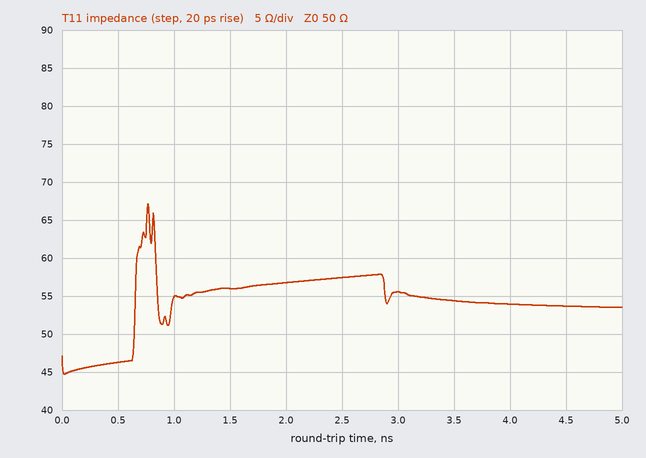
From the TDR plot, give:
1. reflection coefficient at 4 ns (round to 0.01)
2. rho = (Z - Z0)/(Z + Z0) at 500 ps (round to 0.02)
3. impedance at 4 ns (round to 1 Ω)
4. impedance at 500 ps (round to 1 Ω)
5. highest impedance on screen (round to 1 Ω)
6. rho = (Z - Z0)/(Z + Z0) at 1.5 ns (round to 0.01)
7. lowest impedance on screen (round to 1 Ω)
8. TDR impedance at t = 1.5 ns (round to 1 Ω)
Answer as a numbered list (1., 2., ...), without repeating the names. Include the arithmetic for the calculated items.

1. (54 − 50)/(54 + 50) ≈ +0.04
2. (46 − 50)/(46 + 50) ≈ -0.04
3. 54 Ω
4. 46 Ω
5. 67 Ω
6. (56 − 50)/(56 + 50) ≈ +0.06
7. 45 Ω
8. 56 Ω
